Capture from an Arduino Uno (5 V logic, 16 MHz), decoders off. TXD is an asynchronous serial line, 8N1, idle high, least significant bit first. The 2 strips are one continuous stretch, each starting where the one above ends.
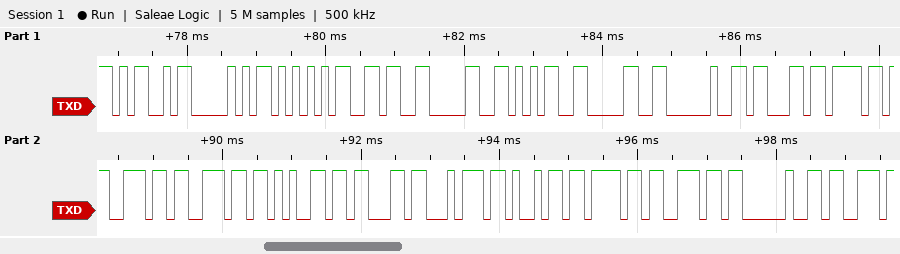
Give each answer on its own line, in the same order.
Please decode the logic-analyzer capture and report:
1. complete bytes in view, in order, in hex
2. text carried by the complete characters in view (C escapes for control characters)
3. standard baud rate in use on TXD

4D 50 55 36 30 35 30 20 63 6F 6E 6E 65 63 74 69 6F 6E 20 73
"MPU6050 connection s"
9600 baud
